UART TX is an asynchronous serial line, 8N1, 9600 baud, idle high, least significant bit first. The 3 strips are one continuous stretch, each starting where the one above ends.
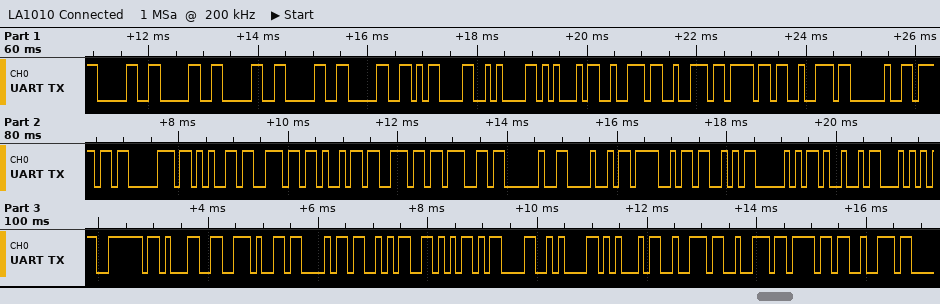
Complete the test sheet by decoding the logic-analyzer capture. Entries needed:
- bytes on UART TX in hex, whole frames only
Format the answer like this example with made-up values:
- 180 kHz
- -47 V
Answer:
- 30 30 30 30 30 0D 0A 45 72 72 6F 72 20 6F 70 65 6E 69 6E 67 20 48 4F 53 50 49 54 7E 31 2E 43 53 56 0D 0A 45 72 72 6F 72
